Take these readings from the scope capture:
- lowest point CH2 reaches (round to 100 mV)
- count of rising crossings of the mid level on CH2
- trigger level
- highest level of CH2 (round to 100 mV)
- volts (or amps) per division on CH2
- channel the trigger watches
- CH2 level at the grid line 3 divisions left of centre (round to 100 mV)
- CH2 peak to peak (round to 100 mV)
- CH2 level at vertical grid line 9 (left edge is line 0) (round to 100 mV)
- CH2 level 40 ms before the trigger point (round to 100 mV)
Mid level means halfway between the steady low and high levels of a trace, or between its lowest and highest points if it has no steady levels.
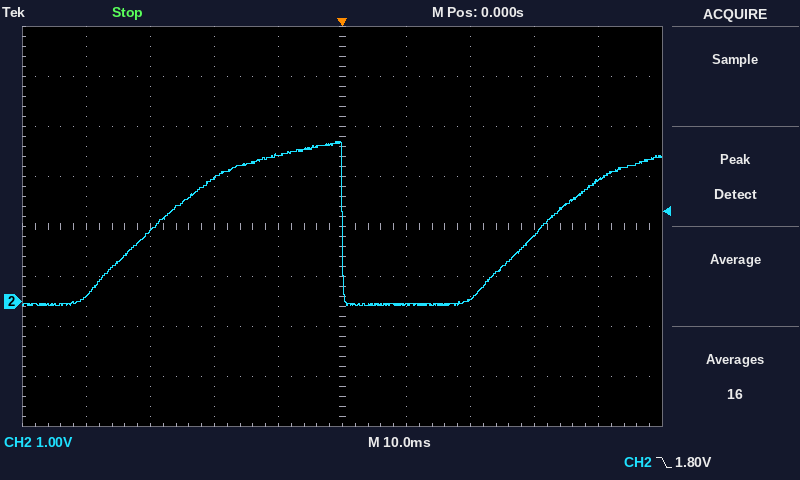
-100 mV
2
1.80 V
3.2 V
1 V
CH2
1.4 V
3.3 V
2.4 V
100 mV
